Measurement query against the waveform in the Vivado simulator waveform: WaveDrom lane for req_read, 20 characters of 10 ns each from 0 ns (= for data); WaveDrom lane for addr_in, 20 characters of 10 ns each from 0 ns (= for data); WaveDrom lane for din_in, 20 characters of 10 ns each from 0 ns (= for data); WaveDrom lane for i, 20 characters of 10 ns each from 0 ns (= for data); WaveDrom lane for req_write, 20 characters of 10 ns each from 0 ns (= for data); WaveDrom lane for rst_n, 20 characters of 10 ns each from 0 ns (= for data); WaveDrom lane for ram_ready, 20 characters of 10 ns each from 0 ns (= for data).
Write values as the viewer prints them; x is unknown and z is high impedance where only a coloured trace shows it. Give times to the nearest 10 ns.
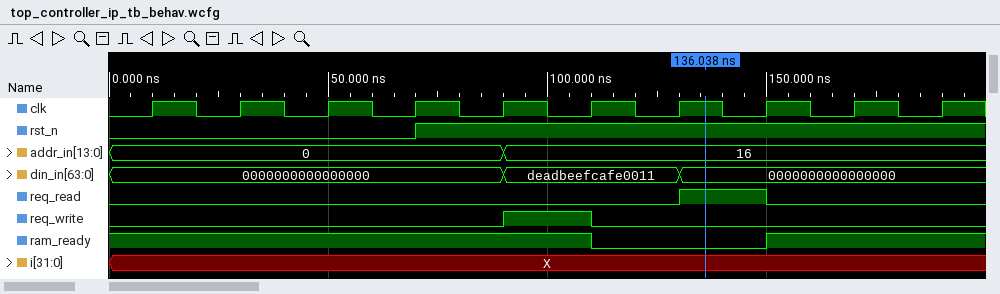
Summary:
{name: 'req_read', wave: '0............1.0....'}
{name: 'addr_in', wave: '=........=..........', data: '0 16'}
{name: 'din_in', wave: '=........=...=......', data: '0000000000000000 deadbeefcafe0011 0000000000000000'}
{name: 'i', wave: 'x...................'}
{name: 'req_write', wave: '0........1.0........'}
{name: 'rst_n', wave: '0......1............'}
{name: 'ram_ready', wave: '1..........0...1....'}
